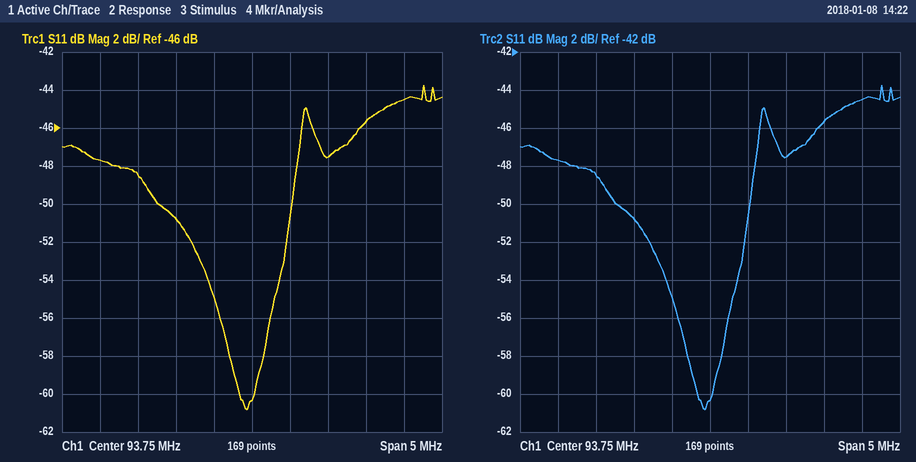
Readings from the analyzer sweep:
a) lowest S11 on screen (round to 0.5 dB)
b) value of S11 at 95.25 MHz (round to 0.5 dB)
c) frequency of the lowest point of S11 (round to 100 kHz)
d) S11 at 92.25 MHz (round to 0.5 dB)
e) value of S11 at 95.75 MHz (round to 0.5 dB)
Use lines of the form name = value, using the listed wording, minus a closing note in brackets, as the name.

lowest S11 on screen = -61.0 dB
value of S11 at 95.25 MHz = -45.5 dB
frequency of the lowest point of S11 = 93.7 MHz
S11 at 92.25 MHz = -48.5 dB
value of S11 at 95.75 MHz = -44.5 dB
